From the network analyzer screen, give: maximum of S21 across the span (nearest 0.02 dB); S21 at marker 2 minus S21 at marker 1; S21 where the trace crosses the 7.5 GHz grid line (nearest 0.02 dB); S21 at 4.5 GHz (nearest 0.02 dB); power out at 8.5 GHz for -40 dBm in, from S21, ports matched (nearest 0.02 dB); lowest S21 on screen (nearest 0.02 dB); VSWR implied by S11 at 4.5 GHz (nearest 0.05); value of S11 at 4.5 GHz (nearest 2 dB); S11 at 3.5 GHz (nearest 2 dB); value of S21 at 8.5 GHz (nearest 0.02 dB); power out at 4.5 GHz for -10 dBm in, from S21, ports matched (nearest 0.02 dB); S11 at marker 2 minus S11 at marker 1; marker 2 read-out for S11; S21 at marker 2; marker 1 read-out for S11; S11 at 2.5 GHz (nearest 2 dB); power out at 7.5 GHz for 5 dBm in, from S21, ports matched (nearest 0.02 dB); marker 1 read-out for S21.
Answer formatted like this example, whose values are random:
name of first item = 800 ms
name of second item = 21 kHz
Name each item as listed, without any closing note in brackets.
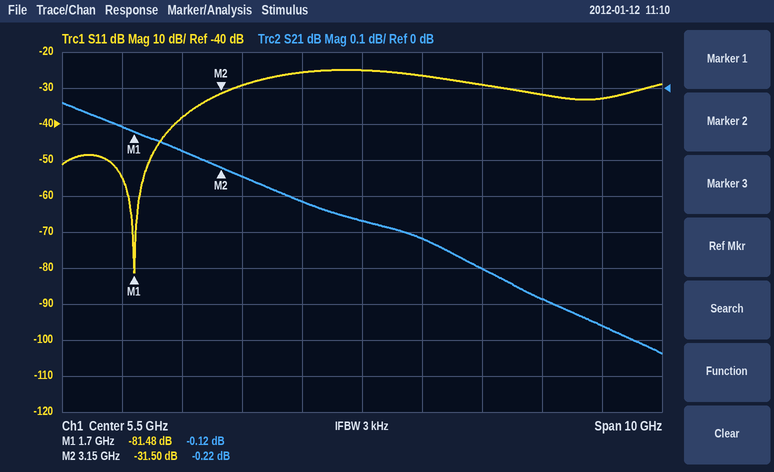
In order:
maximum of S21 across the span = -0.04 dB
S21 at marker 2 minus S21 at marker 1 = -0.10 dB
S21 where the trace crosses the 7.5 GHz grid line = -0.50 dB
S21 at 4.5 GHz = -0.32 dB
power out at 8.5 GHz for -40 dBm in, from S21, ports matched = -40.58 dBm
lowest S21 on screen = -0.74 dB
VSWR implied by S11 at 4.5 GHz = 1.10
value of S11 at 4.5 GHz = -26 dB
S11 at 3.5 GHz = -30 dB
value of S21 at 8.5 GHz = -0.58 dB
power out at 4.5 GHz for -10 dBm in, from S21, ports matched = -10.32 dBm
S11 at marker 2 minus S11 at marker 1 = 49.98 dB
marker 2 read-out for S11 = -31.50 dB
S21 at marker 2 = -0.22 dB
marker 1 read-out for S11 = -81.48 dB
S11 at 2.5 GHz = -38 dB
power out at 7.5 GHz for 5 dBm in, from S21, ports matched = 4.50 dBm
marker 1 read-out for S21 = -0.12 dB
